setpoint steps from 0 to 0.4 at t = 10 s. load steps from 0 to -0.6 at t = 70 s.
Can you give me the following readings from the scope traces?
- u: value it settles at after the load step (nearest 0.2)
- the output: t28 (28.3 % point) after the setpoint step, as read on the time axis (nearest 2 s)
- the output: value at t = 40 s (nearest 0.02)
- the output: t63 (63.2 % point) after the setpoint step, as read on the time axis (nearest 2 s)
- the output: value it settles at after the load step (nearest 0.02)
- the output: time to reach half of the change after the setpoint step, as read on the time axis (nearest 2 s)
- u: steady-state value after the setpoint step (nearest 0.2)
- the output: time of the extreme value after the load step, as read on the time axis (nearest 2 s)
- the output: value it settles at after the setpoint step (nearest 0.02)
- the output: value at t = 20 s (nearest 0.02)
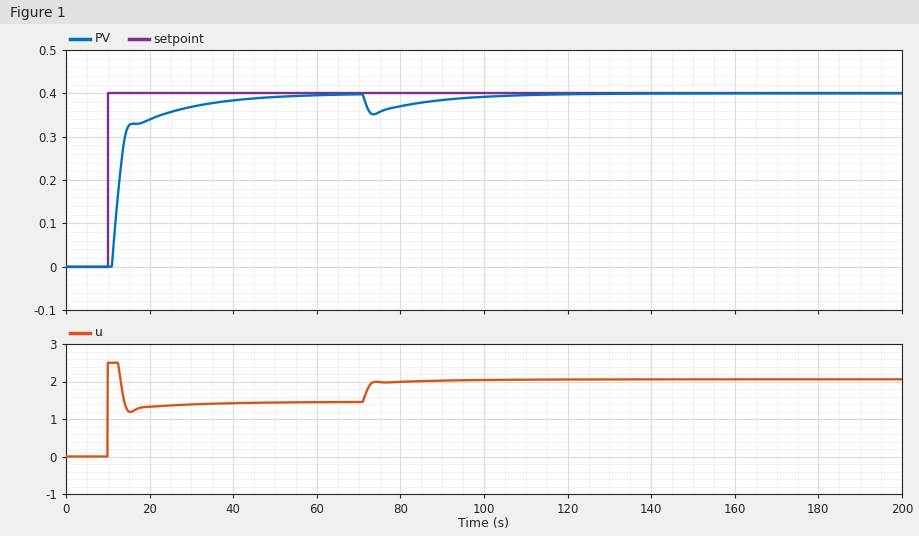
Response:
2.0
12 s
0.38
14 s
0.40
12 s
1.4
74 s
0.40
0.34
